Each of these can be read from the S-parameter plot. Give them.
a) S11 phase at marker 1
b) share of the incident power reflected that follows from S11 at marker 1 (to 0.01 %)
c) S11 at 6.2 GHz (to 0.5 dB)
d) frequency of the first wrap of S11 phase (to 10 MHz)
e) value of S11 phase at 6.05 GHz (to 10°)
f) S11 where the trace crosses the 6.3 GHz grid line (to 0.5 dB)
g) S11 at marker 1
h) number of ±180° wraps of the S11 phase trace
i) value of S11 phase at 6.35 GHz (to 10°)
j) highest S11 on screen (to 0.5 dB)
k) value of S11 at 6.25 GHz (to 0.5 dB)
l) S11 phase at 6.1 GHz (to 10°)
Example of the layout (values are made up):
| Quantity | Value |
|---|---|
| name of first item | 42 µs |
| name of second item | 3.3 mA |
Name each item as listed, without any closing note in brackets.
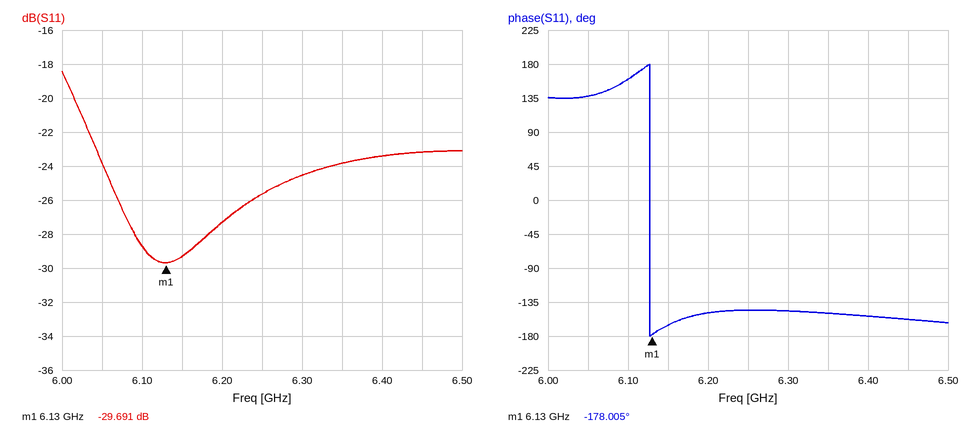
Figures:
| Quantity | Value |
|---|---|
| S11 phase at marker 1 | -178.005° |
| share of the incident power reflected that follows from S11 at marker 1 | 0.11 % |
| S11 at 6.2 GHz | -27.5 dB |
| frequency of the first wrap of S11 phase | 6.13 GHz |
| value of S11 phase at 6.05 GHz | 140° |
| S11 where the trace crosses the 6.3 GHz grid line | -24.5 dB |
| S11 at marker 1 | -29.691 dB |
| number of ±180° wraps of the S11 phase trace | 1 |
| value of S11 phase at 6.35 GHz | -150° |
| highest S11 on screen | -18.5 dB |
| value of S11 at 6.25 GHz | -25.5 dB |
| S11 phase at 6.1 GHz | 160° |
